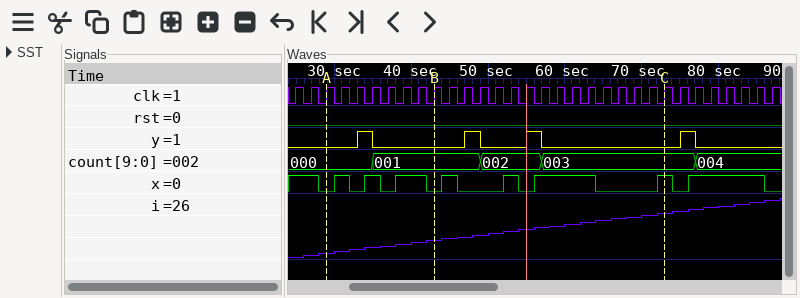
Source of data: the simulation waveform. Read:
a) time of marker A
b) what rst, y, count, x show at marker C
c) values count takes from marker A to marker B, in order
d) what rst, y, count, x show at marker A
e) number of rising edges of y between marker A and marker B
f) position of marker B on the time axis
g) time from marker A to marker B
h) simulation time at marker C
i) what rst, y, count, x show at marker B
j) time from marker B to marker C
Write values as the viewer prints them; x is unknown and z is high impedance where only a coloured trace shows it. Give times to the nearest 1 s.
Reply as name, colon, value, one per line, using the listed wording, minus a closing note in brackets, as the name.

time of marker A: 29 s
what rst, y, count, x show at marker C: rst=0, y=0, count=003, x=1
values count takes from marker A to marker B, in order: 000, 001
what rst, y, count, x show at marker A: rst=0, y=0, count=000, x=0
number of rising edges of y between marker A and marker B: 1
position of marker B on the time axis: 43 s
time from marker A to marker B: 14 s
simulation time at marker C: 73 s
what rst, y, count, x show at marker B: rst=0, y=0, count=001, x=0
time from marker B to marker C: 30 s
